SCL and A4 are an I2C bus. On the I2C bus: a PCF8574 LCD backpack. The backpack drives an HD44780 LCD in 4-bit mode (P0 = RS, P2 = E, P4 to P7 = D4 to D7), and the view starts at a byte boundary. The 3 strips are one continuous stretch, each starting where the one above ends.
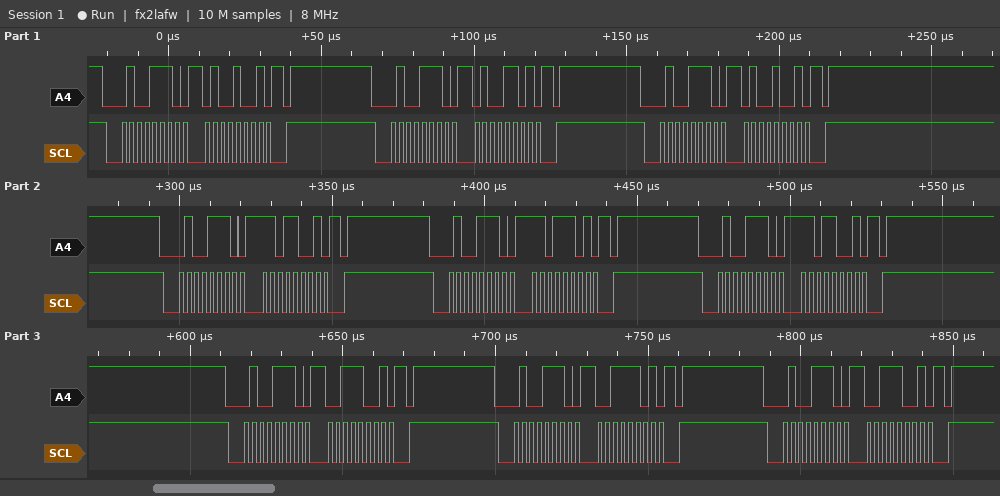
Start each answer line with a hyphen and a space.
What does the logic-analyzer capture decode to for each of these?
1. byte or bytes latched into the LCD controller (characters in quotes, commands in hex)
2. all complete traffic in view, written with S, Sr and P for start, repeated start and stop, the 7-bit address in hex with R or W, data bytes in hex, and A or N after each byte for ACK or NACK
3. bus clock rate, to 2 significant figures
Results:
- 'M'
- S 27W A 49 A P S 27W A 4D A P S 27W A 49 A P S 27W A D9 A P S 27W A DD A P S 27W A D9 A P S 27W A 39 A P S 27W A 3D A P S 27W A 39 A P
- 400 kHz
